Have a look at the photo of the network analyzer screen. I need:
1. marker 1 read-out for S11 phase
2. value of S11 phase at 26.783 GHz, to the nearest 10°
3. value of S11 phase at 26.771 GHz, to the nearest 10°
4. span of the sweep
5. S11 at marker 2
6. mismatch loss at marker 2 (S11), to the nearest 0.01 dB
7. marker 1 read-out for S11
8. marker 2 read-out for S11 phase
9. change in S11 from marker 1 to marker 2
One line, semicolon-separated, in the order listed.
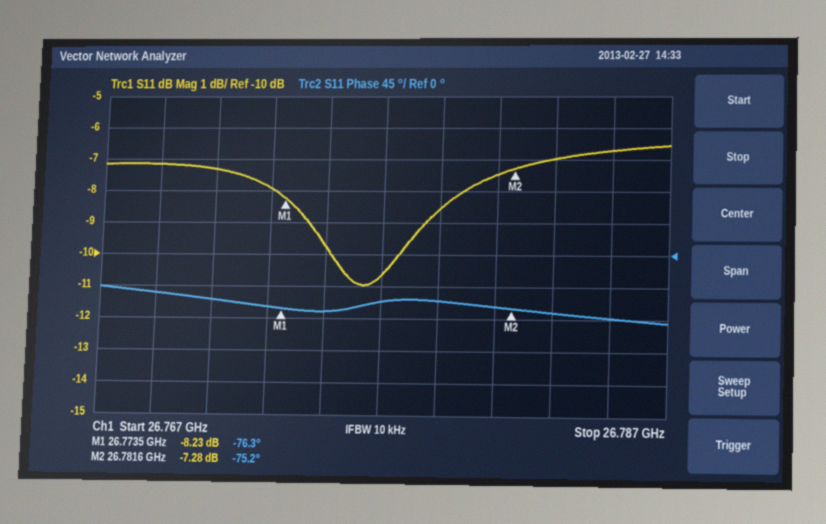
-76.3°; -80°; -60°; 20 MHz; -7.28 dB; 0.90 dB; -8.23 dB; -75.2°; 0.95 dB
